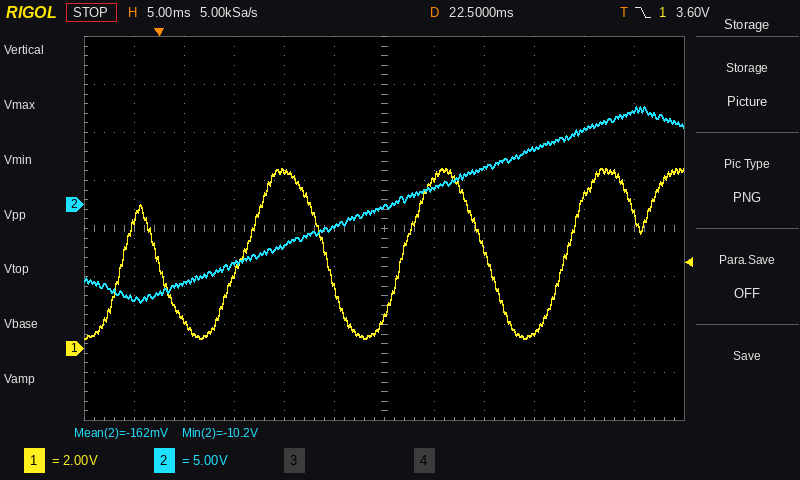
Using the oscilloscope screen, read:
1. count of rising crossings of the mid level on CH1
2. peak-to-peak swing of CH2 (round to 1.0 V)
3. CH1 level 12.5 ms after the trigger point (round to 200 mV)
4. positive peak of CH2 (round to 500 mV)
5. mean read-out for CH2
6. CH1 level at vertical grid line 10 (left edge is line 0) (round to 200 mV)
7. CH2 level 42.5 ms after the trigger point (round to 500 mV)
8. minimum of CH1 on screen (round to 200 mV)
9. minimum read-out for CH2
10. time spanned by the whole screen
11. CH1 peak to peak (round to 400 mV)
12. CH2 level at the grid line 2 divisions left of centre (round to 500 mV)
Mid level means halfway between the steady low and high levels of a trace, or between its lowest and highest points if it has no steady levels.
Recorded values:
4
20.0 V
7.4 V
10.0 V
-162 mV
6.4 V
8.0 V
400 mV
-10.2 V
60 ms
7.2 V
-4.5 V
